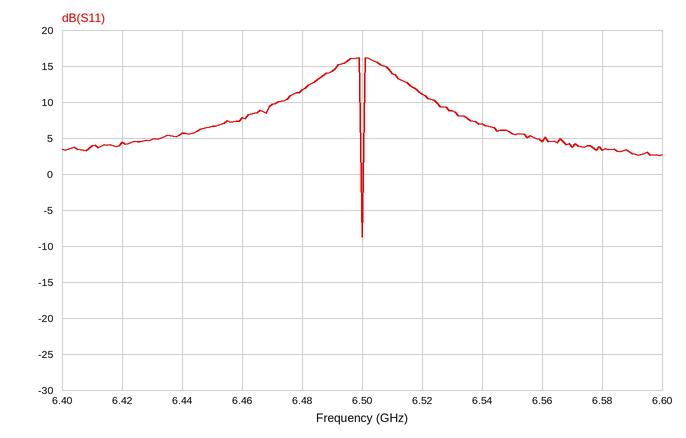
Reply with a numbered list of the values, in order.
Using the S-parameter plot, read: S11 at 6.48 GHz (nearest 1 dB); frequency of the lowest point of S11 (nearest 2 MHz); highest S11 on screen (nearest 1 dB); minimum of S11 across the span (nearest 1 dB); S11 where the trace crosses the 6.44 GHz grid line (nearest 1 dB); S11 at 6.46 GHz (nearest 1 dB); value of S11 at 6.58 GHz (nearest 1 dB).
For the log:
1. 12 dB
2. 6.500 GHz
3. 16 dB
4. -9 dB
5. 6 dB
6. 8 dB
7. 3 dB
